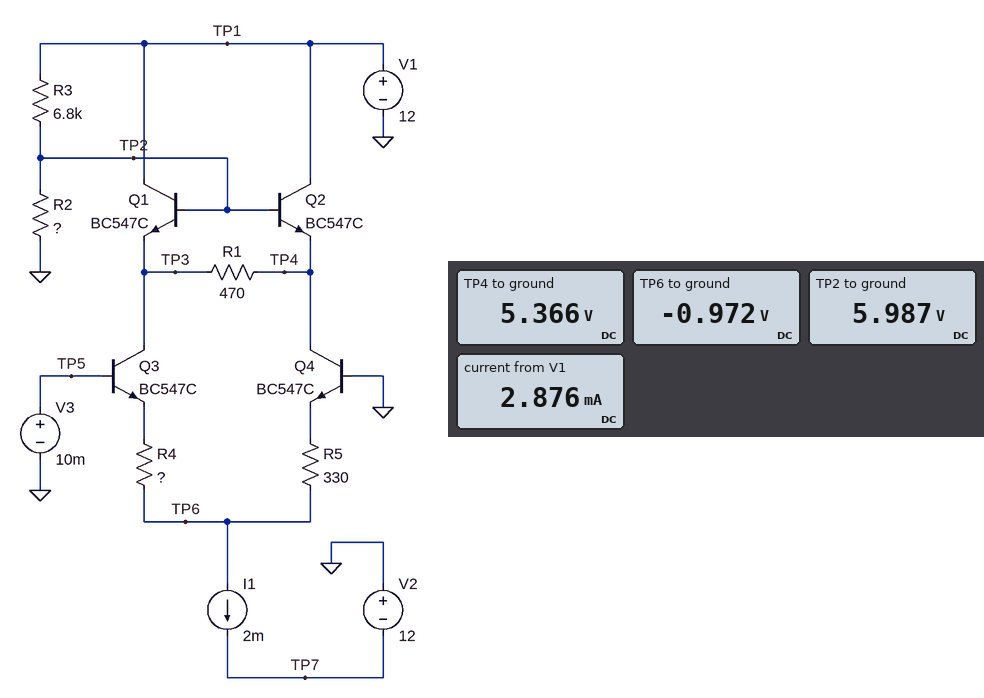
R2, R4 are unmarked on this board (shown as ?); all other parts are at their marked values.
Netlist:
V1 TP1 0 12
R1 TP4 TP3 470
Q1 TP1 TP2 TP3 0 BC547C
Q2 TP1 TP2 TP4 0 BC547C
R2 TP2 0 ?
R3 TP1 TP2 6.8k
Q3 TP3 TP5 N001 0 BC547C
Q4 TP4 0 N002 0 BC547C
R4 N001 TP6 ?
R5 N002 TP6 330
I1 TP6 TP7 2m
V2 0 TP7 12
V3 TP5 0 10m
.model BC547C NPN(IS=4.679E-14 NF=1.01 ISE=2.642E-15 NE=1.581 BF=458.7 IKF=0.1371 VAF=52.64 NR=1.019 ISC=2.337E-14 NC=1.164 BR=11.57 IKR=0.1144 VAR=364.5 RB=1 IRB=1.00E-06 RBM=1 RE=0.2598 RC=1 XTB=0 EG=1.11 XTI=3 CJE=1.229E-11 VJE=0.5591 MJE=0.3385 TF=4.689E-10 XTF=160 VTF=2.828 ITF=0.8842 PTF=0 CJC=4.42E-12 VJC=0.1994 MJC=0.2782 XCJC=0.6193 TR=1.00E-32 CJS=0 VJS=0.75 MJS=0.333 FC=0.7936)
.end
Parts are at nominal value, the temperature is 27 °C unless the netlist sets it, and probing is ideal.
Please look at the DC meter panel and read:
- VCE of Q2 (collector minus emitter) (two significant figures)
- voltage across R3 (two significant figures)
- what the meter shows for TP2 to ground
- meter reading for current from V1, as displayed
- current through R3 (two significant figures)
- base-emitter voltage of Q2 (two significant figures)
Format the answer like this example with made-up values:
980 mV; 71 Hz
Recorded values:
6.6 V; 6.0 V; 5.987 V; 2.876 mA; 880 µA; 620 mV
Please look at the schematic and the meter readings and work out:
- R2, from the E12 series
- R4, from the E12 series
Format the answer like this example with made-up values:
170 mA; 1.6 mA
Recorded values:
6.8 kΩ; 390 Ω
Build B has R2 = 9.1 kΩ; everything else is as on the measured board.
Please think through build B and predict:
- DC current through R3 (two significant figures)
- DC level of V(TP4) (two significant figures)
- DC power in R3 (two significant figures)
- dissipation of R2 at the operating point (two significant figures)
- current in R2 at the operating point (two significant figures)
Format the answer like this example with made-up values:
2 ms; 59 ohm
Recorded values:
760 µA; 6.2 V; 3.9 mW; 5.2 mW; 750 µA
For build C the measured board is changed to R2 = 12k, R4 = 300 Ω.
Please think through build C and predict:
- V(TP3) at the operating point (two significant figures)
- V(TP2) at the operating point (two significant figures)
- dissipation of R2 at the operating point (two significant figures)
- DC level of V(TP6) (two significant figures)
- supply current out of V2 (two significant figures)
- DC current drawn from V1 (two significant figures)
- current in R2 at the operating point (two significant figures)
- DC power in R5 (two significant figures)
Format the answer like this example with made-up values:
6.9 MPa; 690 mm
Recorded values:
7.0 V; 7.6 V; 4.9 mW; -930 mV; 2.0 mA; 2.6 mA; 640 µA; 290 µW
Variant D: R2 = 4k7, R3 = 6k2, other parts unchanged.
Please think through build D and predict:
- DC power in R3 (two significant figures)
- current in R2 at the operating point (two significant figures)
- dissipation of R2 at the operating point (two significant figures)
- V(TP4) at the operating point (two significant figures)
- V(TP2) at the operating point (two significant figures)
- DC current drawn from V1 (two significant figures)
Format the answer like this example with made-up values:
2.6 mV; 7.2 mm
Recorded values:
7.5 mW; 1.1 mA; 5.7 mW; 4.5 V; 5.2 V; 3.1 mA
